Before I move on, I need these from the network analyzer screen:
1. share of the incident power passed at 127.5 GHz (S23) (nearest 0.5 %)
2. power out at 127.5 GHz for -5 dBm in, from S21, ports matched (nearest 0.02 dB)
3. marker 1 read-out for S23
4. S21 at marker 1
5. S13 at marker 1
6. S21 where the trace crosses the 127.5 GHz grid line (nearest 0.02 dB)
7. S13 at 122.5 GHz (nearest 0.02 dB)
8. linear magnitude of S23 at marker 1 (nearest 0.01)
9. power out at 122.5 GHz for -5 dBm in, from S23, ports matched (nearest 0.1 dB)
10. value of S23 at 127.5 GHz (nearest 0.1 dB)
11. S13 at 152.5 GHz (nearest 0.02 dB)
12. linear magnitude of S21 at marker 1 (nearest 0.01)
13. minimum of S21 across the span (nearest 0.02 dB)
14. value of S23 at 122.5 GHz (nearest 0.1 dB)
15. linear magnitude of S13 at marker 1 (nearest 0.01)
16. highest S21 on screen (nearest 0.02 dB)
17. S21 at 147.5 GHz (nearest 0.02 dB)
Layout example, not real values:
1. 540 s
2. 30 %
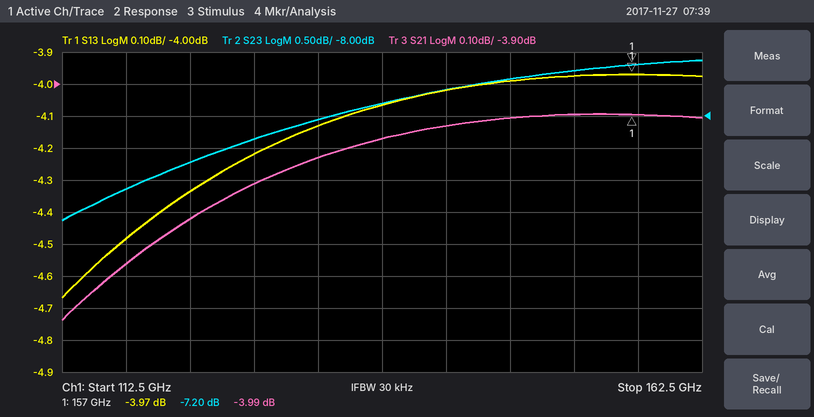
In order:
1. 14.5 %
2. -9.22 dBm
3. -7.20 dB
4. -3.99 dB
5. -3.97 dB
6. -4.22 dB
7. -4.34 dB
8. 0.44
9. -13.7 dBm
10. -8.4 dB
11. -3.98 dB
12. 0.63
13. -4.64 dB
14. -8.7 dB
15. 0.63
16. -4.00 dB
17. -4.00 dB
